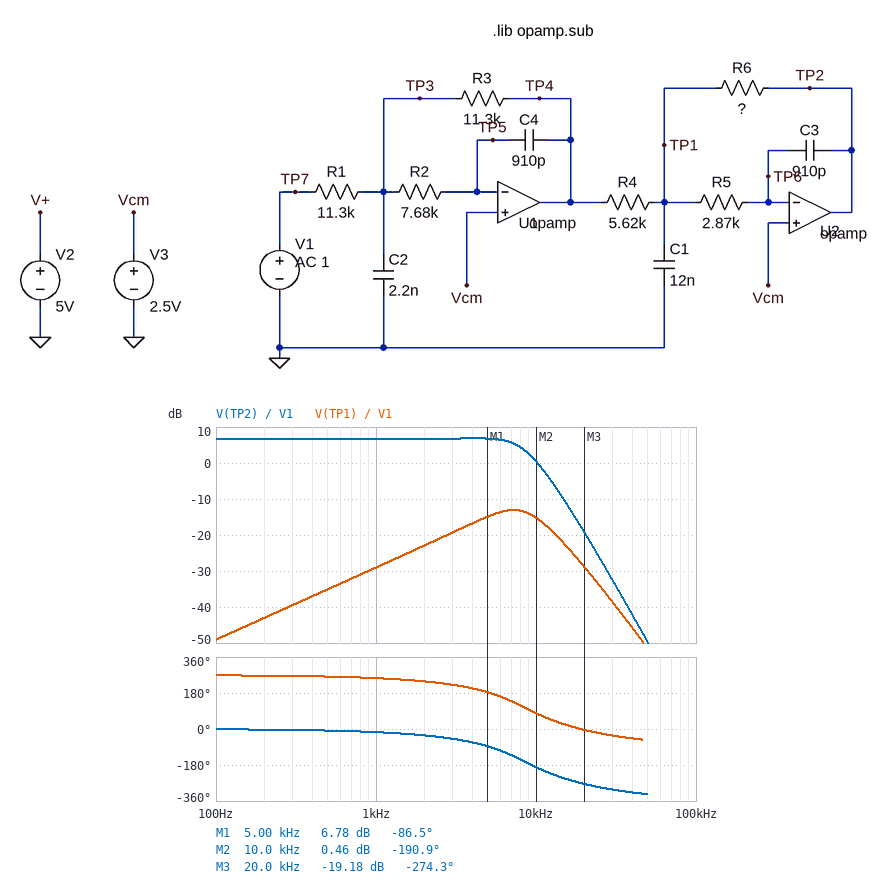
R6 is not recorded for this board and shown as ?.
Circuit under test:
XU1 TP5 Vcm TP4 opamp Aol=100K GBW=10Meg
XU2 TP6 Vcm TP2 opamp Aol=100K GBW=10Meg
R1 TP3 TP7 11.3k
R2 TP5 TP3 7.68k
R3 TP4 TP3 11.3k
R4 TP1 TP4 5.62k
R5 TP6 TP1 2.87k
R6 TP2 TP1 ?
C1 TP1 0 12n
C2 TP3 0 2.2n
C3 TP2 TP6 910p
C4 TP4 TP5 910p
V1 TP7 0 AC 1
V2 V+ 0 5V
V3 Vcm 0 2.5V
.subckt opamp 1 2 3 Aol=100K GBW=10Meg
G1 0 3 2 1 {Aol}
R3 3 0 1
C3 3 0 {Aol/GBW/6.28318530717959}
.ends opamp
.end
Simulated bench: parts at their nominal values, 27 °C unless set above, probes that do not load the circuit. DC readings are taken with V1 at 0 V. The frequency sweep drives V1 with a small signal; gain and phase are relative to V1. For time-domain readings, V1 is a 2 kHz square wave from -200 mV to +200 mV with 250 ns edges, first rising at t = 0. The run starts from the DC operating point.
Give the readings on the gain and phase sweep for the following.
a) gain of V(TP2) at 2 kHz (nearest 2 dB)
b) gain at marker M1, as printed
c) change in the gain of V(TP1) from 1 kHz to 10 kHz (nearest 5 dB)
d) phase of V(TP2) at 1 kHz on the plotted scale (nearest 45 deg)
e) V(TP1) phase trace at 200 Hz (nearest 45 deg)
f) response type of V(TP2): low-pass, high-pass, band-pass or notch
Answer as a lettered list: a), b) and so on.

a) 6 dB
b) 6.78 dB
c) 15 dB
d) 0 deg
e) 270 deg
f) low-pass
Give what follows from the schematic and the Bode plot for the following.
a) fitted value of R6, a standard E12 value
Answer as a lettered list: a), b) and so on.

a) 12 kΩ
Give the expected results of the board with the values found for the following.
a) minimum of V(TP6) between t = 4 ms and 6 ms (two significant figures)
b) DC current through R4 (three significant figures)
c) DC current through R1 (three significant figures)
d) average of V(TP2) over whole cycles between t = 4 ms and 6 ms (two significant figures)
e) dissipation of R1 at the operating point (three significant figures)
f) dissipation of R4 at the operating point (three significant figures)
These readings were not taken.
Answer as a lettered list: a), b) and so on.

a) 2.5 V
b) 445 µA
c) 221 µA
d) -2.8 V
e) 553 µW
f) 1.11 mW
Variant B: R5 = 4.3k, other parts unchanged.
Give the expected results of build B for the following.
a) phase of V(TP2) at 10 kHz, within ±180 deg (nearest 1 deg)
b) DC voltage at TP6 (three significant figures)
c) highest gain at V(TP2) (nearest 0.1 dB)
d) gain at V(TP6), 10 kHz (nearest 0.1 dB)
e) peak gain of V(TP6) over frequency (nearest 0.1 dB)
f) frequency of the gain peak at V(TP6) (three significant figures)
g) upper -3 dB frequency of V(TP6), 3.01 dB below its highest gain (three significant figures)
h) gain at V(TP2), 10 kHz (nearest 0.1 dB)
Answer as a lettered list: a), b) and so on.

a) 151 deg
b) 2.50 V
c) 7.2 dB
d) -62.9 dB
e) -58.4 dB
f) 6.15 kHz
g) 9.07 kHz
h) -2.9 dB
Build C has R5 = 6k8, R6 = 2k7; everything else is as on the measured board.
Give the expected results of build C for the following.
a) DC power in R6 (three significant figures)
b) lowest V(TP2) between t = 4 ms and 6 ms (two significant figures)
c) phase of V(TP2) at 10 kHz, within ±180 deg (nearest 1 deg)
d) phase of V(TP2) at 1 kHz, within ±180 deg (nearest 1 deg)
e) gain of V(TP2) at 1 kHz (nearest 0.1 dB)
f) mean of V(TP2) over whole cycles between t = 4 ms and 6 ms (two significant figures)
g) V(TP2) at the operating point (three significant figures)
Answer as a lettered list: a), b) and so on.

a) 534 µW
b) 1.2 V
c) -153 deg
d) -13 deg
e) -6.4 dB
f) 1.3 V
g) 1.30 V
